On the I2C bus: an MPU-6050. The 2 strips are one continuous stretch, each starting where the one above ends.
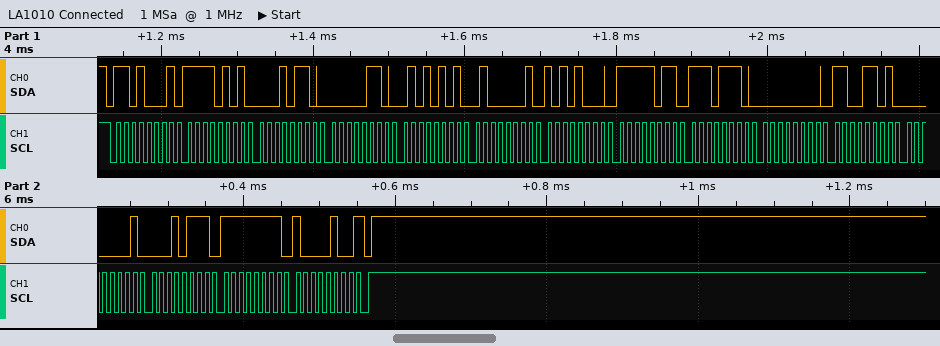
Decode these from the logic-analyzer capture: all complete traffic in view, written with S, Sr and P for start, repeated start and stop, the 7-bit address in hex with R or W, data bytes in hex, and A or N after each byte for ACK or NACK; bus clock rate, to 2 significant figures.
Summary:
S 68R A F5 A 16 A 06 A 55 A 41 A A8 A FB A EE A 00 A CD A 01 A 17 A FF A 84 N P
100 kHz
